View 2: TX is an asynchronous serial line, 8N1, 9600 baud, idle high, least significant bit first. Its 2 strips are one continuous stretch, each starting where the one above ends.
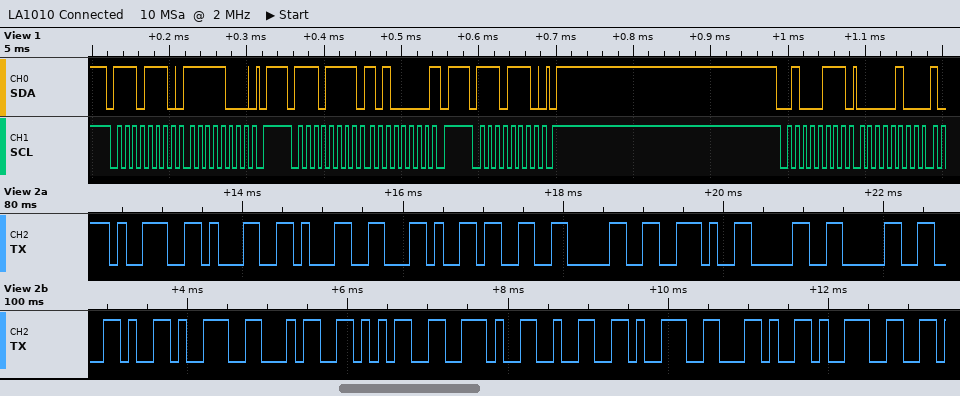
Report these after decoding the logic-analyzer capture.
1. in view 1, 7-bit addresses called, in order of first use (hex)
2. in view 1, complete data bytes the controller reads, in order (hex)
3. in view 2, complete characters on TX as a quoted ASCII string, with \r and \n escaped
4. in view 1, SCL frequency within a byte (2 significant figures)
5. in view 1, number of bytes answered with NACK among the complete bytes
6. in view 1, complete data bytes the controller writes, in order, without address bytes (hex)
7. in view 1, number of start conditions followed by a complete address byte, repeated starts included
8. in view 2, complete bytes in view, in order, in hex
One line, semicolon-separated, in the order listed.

0x77 0x23; A0 04; "911,30.00,945.29,9"; 100 kHz; 1; F8; 4; 39 31 31 2C 33 30 2E 30 30 2C 39 34 35 2E 32 39 2C 39
